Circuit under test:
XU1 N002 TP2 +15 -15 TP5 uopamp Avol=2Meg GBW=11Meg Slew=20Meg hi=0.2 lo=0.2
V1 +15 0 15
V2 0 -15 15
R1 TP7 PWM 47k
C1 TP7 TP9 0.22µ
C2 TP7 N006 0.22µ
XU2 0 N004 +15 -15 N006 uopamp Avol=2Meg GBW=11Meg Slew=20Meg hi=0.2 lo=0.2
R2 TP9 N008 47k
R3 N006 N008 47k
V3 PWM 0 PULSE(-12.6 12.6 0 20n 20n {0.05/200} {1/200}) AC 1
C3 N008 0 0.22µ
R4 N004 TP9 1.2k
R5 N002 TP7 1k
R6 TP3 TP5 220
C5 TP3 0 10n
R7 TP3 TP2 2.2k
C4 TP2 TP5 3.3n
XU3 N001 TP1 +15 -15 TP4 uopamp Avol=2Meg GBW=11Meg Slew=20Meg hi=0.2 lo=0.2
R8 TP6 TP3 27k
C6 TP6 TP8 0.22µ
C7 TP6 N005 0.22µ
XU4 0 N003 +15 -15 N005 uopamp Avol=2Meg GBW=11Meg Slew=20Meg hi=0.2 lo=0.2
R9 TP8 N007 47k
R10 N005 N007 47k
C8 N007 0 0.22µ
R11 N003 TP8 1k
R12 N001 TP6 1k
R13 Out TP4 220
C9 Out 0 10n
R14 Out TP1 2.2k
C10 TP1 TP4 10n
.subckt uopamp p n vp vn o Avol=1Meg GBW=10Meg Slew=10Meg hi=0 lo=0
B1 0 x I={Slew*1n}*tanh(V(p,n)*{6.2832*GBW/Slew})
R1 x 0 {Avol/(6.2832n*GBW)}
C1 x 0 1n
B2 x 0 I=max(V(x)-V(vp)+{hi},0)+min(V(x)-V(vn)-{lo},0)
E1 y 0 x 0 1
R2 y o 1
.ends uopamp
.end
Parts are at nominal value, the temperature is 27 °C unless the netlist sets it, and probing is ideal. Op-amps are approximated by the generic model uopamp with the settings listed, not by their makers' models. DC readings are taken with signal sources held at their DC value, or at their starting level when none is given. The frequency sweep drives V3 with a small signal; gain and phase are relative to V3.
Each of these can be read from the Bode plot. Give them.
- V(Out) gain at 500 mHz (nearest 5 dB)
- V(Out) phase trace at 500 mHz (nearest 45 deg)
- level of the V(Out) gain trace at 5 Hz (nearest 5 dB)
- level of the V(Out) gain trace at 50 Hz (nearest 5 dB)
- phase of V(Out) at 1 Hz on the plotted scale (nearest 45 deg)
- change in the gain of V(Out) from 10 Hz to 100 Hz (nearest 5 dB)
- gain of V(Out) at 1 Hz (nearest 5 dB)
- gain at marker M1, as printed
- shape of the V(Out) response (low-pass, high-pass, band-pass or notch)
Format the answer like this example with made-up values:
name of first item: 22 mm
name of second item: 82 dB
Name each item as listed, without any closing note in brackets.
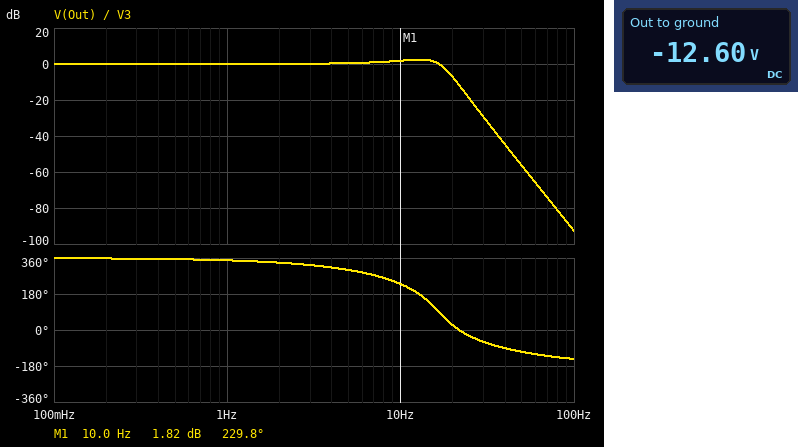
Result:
V(Out) gain at 500 mHz: 0 dB
V(Out) phase trace at 500 mHz: 360 deg
level of the V(Out) gain trace at 5 Hz: 0 dB
level of the V(Out) gain trace at 50 Hz: -55 dB
phase of V(Out) at 1 Hz on the plotted scale: 360 deg
change in the gain of V(Out) from 10 Hz to 100 Hz: -95 dB
gain of V(Out) at 1 Hz: 0 dB
gain at marker M1, as printed: 1.82 dB
shape of the V(Out) response: low-pass
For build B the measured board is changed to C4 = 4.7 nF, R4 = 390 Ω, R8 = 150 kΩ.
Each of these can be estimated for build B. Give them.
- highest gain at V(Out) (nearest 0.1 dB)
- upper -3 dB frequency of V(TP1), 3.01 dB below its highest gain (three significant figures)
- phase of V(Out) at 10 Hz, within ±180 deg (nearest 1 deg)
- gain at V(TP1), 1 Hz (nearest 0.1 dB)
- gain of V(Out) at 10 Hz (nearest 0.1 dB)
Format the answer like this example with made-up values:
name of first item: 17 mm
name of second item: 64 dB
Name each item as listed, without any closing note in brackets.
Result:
highest gain at V(Out): 0 dB
upper -3 dB frequency of V(TP1), 3.01 dB below its highest gain: 2.91 Hz
phase of V(Out) at 10 Hz, within ±180 deg: 161 deg
gain at V(TP1), 1 Hz: -0.5 dB
gain of V(Out) at 10 Hz: -11.6 dB
